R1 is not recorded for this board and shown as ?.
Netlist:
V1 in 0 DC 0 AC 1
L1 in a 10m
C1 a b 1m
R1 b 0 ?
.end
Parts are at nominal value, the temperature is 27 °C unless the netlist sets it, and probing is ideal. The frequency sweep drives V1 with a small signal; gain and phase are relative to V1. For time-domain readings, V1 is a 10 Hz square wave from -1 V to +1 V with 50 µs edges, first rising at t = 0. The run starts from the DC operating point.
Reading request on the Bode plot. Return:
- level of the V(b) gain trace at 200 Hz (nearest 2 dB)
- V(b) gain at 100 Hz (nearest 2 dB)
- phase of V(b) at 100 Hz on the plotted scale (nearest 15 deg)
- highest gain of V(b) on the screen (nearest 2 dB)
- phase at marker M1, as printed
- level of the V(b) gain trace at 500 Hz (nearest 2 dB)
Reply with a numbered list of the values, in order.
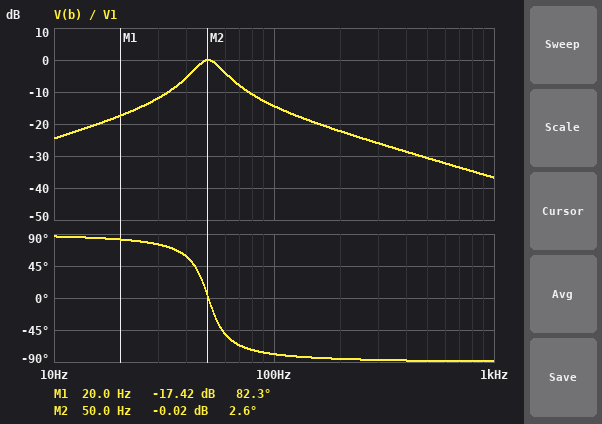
1. -22 dB
2. -14 dB
3. -75 deg
4. 0 dB
5. 82.3 deg
6. -30 dB
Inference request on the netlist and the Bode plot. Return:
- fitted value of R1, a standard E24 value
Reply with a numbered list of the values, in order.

1. 0.91 Ω
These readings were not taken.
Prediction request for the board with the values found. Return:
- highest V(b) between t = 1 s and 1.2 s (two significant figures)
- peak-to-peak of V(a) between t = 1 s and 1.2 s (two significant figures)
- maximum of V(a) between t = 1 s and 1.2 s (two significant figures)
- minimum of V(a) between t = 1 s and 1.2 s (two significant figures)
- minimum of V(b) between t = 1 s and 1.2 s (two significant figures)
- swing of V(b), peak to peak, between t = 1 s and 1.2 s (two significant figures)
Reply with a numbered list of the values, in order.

1. 520 mV
2. 4.9 V
3. 2.5 V
4. -2.5 V
5. -520 mV
6. 1.0 V
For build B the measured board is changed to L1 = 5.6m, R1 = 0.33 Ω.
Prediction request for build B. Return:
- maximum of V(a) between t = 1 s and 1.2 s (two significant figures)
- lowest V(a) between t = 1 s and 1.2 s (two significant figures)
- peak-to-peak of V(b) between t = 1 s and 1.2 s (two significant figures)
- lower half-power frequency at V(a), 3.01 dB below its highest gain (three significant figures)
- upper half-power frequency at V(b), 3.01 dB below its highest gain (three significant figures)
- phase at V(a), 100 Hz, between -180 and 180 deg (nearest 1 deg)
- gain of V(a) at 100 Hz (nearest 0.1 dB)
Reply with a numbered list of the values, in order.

1. 2.8 V
2. -2.8 V
3. 560 mV
4. 62.1 Hz
5. 72.1 Hz
6. -159 deg
7. -1.6 dB
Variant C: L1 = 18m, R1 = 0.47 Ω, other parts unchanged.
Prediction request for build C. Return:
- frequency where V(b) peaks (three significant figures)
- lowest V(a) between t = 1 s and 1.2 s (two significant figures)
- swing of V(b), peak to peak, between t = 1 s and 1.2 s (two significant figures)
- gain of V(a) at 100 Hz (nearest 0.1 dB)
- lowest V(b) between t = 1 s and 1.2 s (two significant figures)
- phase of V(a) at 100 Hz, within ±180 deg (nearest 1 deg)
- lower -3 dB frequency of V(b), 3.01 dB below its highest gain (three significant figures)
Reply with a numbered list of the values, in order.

1. 37.5 Hz
2. -2.2 V
3. 290 mV
4. -15.4 dB
5. -150 mV
6. -161 deg
7. 35.5 Hz
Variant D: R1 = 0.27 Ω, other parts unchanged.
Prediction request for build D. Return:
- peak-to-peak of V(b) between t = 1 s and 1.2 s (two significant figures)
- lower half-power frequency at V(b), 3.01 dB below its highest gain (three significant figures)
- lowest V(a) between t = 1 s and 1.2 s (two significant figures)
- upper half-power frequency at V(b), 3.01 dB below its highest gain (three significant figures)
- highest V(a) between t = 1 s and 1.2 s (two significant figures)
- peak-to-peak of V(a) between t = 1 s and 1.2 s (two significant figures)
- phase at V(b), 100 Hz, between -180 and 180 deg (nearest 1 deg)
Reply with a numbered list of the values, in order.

1. 650 mV
2. 48.2 Hz
3. -4.6 V
4. 52.5 Hz
5. 4.6 V
6. 9.1 V
7. -87 deg
